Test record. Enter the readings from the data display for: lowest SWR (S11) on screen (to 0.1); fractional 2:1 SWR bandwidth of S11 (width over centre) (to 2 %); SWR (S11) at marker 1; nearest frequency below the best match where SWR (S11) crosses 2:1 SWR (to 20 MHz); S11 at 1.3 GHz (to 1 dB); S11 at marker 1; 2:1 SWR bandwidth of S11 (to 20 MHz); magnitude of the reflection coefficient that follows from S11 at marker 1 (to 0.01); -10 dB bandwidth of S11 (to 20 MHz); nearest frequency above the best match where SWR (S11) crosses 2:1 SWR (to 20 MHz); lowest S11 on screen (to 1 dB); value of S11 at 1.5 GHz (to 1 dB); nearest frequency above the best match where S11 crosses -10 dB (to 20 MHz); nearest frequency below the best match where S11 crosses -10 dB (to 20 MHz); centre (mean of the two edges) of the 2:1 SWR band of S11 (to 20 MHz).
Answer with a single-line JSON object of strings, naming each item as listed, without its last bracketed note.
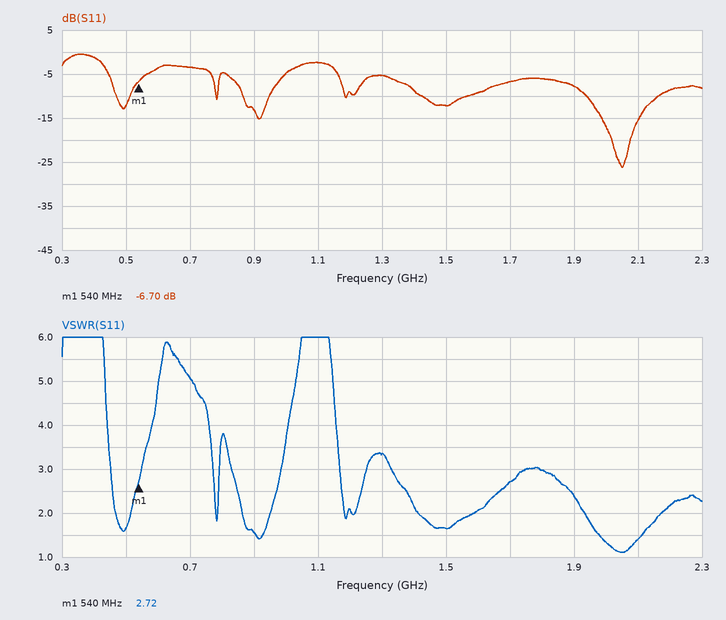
{"lowest SWR (S11) on screen": "1.1", "fractional 2:1 SWR bandwidth of S11 (width over centre)": "12 %", "SWR (S11) at marker 1": "2.72", "nearest frequency below the best match where SWR (S11) crosses 2:1 SWR": "1.94 GHz", "S11 at 1.3 GHz": "-5 dB", "S11 at marker 1": "-6.70 dB", "2:1 SWR bandwidth of S11": "240 MHz", "magnitude of the reflection coefficient that follows from S11 at marker 1": "0.46", "-10 dB bandwidth of S11": "220 MHz", "nearest frequency above the best match where SWR (S11) crosses 2:1 SWR": "2.18 GHz", "lowest S11 on screen": "-26 dB", "value of S11 at 1.5 GHz": "-12 dB", "nearest frequency above the best match where S11 crosses -10 dB": "2.16 GHz", "nearest frequency below the best match where S11 crosses -10 dB": "1.94 GHz", "centre (mean of the two edges) of the 2:1 SWR band of S11": "2.06 GHz"}
